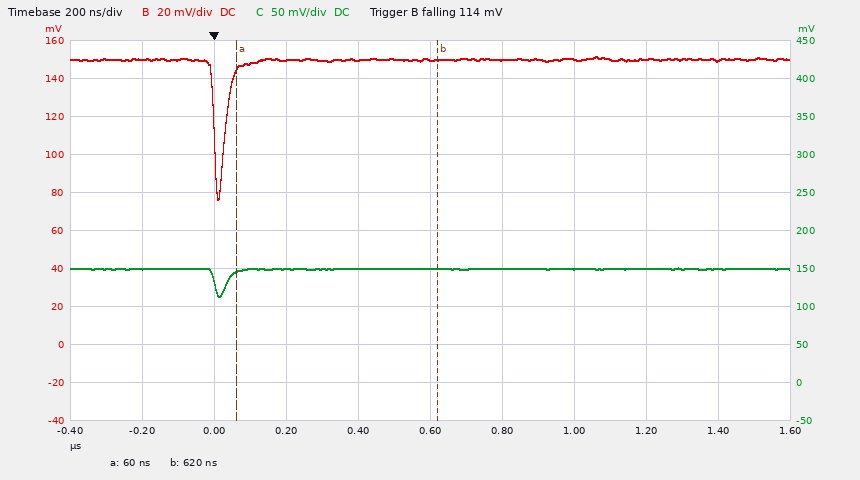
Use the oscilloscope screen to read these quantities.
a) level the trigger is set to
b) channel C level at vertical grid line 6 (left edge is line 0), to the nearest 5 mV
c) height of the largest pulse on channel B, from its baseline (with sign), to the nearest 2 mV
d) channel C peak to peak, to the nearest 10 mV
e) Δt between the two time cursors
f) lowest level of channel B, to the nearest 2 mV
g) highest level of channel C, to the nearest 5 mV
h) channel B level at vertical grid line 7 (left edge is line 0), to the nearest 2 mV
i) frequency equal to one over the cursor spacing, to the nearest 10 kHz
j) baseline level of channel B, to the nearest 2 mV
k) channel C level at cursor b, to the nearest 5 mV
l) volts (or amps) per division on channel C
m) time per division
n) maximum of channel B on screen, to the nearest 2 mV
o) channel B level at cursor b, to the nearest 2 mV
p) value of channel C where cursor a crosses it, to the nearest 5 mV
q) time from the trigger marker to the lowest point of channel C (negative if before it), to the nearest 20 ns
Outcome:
114 mV
150 mV
-74 mV
40 mV
560 ns
76 mV
150 mV
150 mV
1.79 MHz
150 mV
150 mV
50 mV
200 ns
152 mV
150 mV
145 mV
+20 ns
